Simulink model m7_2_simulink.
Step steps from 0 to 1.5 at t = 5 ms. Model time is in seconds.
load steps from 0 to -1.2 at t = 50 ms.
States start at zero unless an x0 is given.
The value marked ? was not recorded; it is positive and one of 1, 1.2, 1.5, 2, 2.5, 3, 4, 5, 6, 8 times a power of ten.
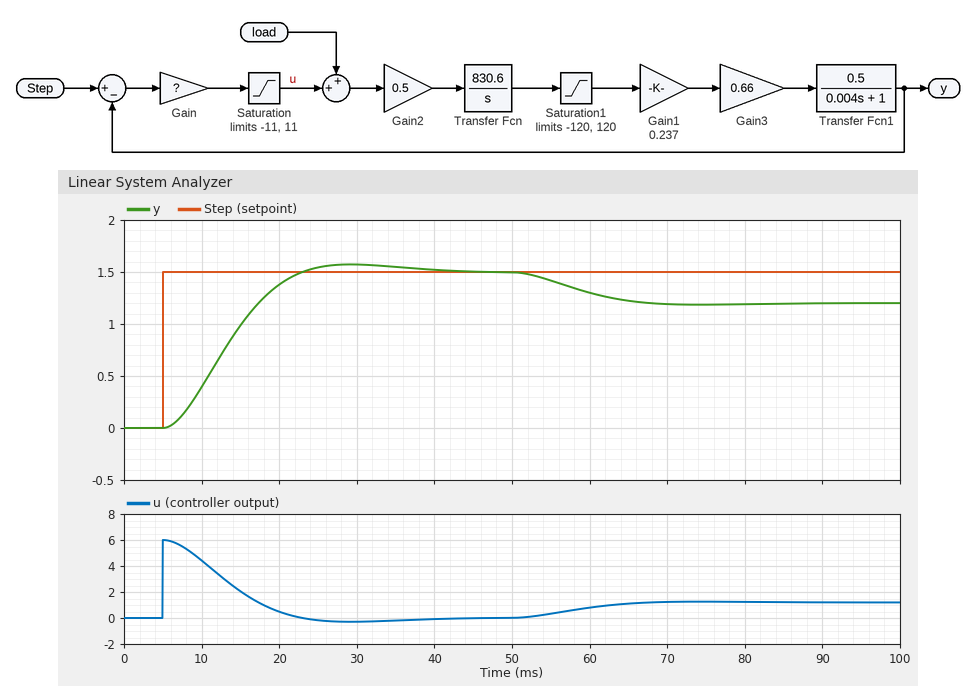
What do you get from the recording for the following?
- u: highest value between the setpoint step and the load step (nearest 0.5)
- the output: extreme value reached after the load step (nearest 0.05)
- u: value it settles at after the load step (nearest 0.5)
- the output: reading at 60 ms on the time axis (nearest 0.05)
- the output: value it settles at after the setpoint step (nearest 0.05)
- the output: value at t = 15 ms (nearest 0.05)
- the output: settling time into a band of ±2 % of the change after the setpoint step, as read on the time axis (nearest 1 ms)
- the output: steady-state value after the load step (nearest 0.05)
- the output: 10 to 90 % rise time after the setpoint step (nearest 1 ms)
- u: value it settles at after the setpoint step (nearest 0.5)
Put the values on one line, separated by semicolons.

6.0; 1.20; 1.0; 1.30; 1.50; 1.00; 38 ms; 1.20; 12 ms; 0.0
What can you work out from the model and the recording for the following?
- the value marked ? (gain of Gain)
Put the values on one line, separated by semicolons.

4
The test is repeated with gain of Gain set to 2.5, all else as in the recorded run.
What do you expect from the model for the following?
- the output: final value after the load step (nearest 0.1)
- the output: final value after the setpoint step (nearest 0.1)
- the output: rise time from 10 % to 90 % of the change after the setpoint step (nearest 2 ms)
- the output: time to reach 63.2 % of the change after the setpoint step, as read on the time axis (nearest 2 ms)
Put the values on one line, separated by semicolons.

1.0; 1.5; 20 ms; 18 ms
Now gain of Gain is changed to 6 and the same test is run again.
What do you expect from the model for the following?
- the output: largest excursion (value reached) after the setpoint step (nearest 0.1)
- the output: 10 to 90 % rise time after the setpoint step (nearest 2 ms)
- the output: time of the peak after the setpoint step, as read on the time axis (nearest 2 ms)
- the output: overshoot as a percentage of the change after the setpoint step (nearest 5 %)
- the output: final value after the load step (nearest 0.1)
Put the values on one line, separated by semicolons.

1.7; 8 ms; 22 ms; 10 %; 1.3
